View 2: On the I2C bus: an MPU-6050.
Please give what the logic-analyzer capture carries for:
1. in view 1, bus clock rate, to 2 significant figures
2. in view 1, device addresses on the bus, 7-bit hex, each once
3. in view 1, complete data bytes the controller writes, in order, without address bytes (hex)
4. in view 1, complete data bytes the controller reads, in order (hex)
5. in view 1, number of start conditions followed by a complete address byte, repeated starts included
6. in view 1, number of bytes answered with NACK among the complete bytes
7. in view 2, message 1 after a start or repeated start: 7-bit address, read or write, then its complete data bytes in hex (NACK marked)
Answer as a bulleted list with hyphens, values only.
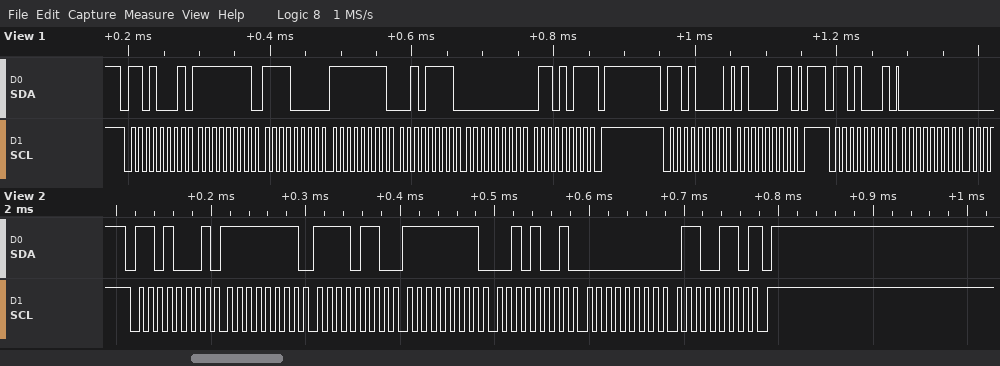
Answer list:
- 100 kHz
- 0x68
- 43
- FF F0 FF 2F 00 6B 00
- 3
- 1
- 0x68 read: FF F6 FF 29 00 66 NACK
